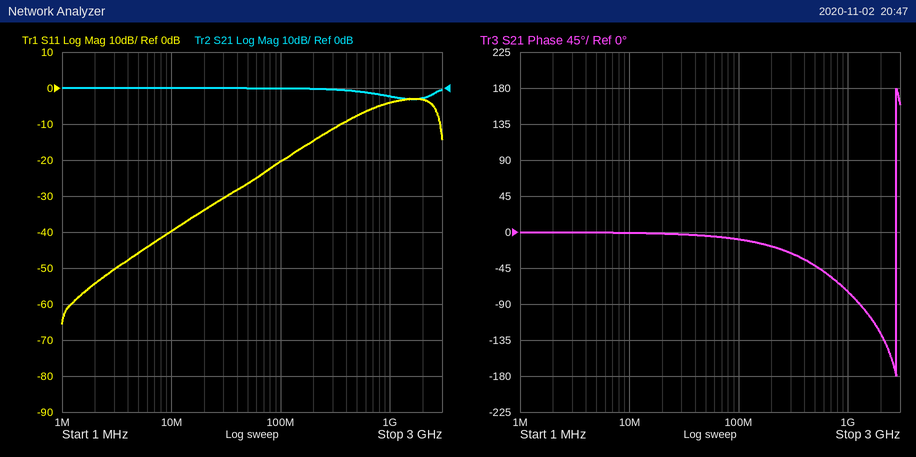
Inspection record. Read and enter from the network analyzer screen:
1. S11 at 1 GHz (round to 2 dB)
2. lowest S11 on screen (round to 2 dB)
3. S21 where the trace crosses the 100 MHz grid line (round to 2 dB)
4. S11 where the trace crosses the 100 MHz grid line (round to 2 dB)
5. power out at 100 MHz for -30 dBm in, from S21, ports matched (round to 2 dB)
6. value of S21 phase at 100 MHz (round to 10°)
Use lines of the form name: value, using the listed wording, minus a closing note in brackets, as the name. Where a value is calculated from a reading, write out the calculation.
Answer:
S11 at 1 GHz: -4 dB
lowest S11 on screen: -66 dB
S21 where the trace crosses the 100 MHz grid line: 0 dB
S11 where the trace crosses the 100 MHz grid line: -20 dB
power out at 100 MHz for -30 dBm in, from S21, ports matched: -30 dBm + (0 dB) = -30 dBm
value of S21 phase at 100 MHz: -10°
